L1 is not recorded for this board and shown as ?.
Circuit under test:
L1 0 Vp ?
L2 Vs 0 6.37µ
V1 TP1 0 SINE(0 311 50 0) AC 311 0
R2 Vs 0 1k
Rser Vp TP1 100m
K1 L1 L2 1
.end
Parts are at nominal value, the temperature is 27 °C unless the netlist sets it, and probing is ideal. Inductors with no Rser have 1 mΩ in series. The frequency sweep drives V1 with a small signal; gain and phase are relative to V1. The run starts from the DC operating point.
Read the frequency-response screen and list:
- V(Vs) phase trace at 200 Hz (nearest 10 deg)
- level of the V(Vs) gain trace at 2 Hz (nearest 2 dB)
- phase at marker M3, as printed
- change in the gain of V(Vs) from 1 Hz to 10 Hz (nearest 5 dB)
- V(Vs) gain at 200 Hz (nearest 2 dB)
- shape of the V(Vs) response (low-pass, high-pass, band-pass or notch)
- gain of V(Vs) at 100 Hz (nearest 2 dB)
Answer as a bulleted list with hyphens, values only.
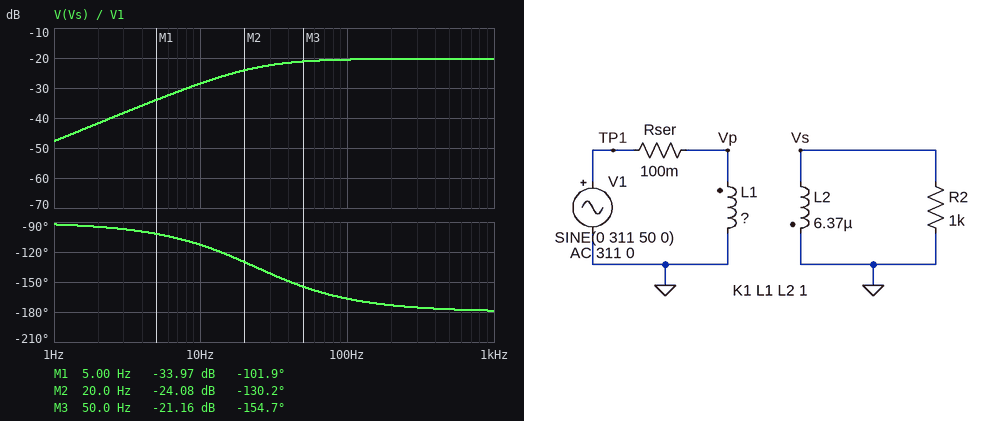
- -170 deg
- -42 dB
- -154.7 deg
- 20 dB
- -20 dB
- high-pass
- -20 dB
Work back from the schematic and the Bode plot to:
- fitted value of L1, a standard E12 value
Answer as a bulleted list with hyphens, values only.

- 680 µH
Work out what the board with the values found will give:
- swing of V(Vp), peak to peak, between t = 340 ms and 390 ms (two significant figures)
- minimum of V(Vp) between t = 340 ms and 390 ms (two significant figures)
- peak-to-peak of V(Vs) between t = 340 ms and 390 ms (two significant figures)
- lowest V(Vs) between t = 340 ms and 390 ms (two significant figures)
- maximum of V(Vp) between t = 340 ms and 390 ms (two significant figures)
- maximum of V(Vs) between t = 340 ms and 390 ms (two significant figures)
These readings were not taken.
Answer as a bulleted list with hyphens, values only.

- 560 V
- -280 V
- 54 V
- -27 V
- 280 V
- 27 V
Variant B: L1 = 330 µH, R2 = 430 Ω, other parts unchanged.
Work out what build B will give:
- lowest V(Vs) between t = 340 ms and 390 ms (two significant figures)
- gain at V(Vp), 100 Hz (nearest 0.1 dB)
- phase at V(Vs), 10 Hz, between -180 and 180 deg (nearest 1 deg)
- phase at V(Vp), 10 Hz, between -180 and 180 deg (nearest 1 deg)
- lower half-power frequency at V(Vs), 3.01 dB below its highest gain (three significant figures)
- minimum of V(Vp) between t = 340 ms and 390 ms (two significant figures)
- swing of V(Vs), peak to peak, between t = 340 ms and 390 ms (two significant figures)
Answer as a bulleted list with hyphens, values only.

- -31 V
- -0.9 dB
- -102 deg
- 76 deg
- 48.7 Hz
- -220 V
- 62 V
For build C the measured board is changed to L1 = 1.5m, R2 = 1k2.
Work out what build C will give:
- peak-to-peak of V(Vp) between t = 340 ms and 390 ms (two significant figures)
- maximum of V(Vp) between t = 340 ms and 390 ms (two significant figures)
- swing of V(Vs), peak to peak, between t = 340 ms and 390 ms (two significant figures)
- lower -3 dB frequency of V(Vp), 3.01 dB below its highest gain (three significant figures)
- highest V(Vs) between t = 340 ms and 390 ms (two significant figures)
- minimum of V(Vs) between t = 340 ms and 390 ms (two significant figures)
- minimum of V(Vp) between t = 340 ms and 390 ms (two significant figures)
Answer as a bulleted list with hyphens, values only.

- 610 V
- 300 V
- 40 V
- 10.7 Hz
- 20 V
- -20 V
- -300 V
